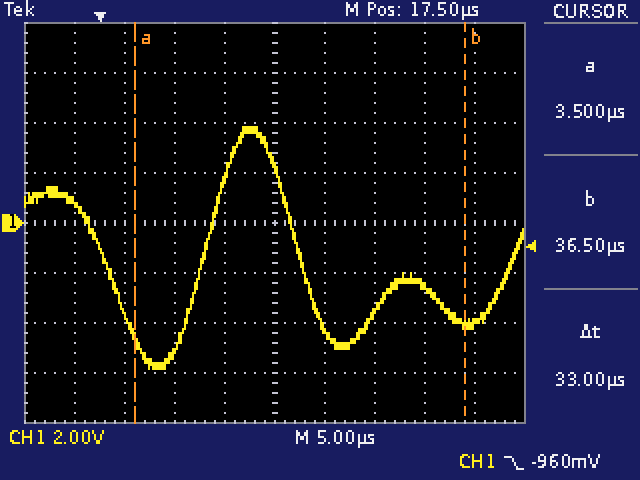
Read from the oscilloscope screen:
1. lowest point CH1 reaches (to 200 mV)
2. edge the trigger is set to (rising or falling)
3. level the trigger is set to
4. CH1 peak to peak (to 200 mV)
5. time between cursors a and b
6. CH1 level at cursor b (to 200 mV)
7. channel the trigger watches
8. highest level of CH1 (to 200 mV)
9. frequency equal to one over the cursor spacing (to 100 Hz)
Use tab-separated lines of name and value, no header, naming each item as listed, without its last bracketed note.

lowest point CH1 reaches	-5.8 V
edge the trigger is set to	falling
level the trigger is set to	-960 mV
CH1 peak to peak	9.6 V
time between cursors a and b	33 µs
CH1 level at cursor b	-4.0 V
channel the trigger watches	CH1
highest level of CH1	3.8 V
frequency equal to one over the cursor spacing	30.3 kHz
